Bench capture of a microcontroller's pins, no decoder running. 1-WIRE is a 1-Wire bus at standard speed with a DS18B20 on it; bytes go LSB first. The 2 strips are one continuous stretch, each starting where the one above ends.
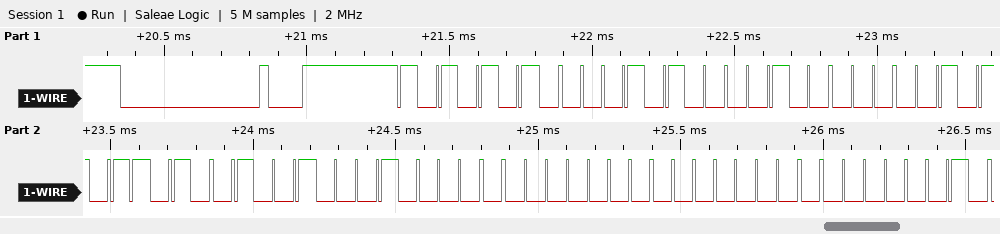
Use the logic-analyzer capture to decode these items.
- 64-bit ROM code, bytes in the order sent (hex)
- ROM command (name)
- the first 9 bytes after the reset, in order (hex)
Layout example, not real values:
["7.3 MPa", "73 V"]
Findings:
["28 04 D4 92 08 00 00 40", "Match ROM", "55 28 04 D4 92 08 00 00 40"]
